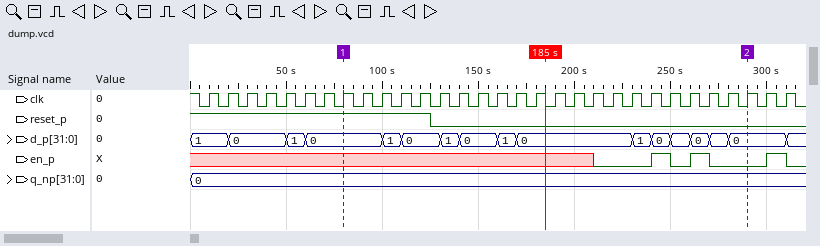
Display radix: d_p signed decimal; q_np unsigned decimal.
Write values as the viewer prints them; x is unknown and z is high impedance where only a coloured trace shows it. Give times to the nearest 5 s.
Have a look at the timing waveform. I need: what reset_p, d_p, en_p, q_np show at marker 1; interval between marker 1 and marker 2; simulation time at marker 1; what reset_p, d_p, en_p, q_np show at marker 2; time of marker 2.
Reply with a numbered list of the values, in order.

1. reset_p=1, d_p=0, en_p=x, q_np=0
2. 210 s
3. 80 s
4. reset_p=0, d_p=0, en_p=0, q_np=0
5. 290 s
